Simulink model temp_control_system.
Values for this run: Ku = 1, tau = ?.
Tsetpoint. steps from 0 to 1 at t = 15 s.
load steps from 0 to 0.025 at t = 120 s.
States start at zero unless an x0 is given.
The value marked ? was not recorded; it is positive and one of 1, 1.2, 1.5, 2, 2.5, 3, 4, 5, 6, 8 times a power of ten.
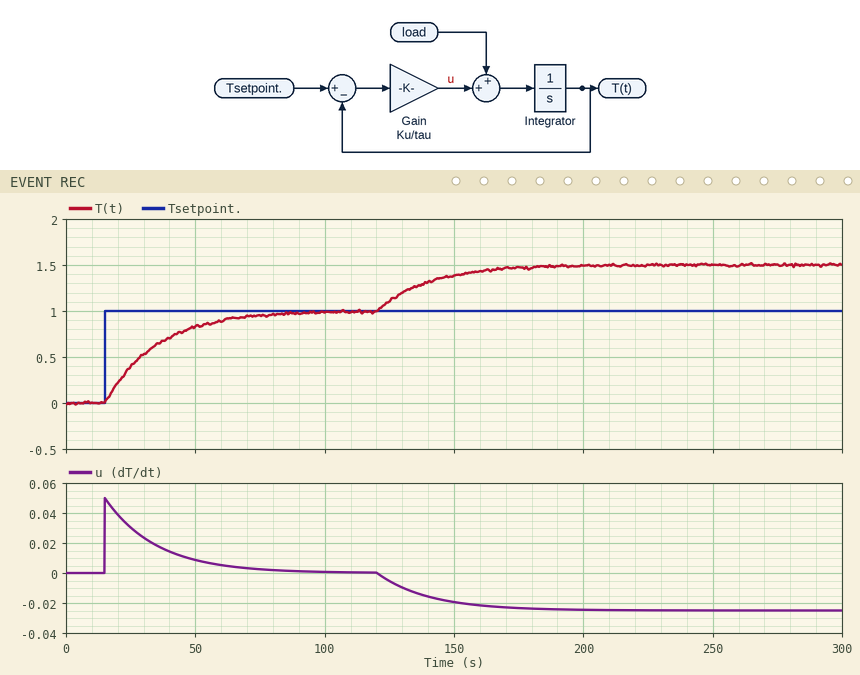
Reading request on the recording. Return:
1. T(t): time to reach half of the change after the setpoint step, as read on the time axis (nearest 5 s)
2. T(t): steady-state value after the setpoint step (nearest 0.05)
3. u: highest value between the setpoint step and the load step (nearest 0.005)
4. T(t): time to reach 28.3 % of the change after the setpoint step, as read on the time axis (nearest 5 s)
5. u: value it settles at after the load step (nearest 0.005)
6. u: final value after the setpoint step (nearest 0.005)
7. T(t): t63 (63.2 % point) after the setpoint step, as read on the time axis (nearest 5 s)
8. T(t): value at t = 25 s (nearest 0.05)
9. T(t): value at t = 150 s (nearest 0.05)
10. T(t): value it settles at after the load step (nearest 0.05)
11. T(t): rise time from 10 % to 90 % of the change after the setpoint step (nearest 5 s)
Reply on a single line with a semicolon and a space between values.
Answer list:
30 s; 1.00; 0.050; 20 s; -0.025; 0.000; 35 s; 0.40; 1.40; 1.50; 45 s
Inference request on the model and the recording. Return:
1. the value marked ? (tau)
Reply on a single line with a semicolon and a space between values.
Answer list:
20
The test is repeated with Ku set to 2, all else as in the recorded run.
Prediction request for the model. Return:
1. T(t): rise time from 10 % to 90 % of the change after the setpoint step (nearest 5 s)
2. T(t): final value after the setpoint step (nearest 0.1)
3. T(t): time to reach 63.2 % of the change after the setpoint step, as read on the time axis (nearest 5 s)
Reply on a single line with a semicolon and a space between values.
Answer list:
20 s; 1.0; 25 s
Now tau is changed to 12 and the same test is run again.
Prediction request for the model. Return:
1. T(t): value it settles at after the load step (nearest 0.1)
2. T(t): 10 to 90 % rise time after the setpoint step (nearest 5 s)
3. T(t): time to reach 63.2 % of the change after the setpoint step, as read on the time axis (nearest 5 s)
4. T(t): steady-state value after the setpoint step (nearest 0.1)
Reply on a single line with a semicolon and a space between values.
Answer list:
1.3; 25 s; 25 s; 1.0
